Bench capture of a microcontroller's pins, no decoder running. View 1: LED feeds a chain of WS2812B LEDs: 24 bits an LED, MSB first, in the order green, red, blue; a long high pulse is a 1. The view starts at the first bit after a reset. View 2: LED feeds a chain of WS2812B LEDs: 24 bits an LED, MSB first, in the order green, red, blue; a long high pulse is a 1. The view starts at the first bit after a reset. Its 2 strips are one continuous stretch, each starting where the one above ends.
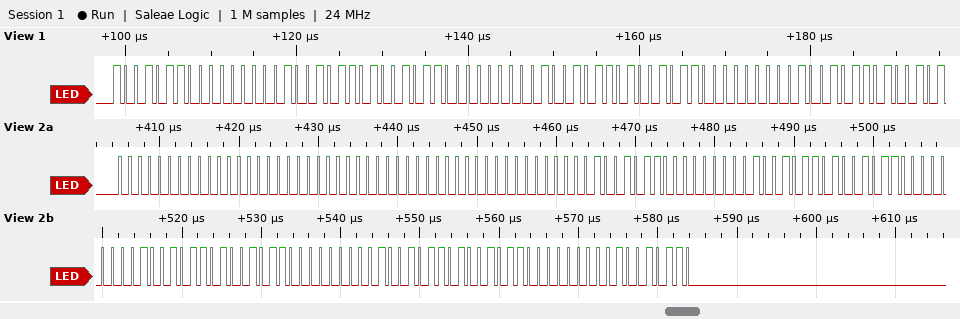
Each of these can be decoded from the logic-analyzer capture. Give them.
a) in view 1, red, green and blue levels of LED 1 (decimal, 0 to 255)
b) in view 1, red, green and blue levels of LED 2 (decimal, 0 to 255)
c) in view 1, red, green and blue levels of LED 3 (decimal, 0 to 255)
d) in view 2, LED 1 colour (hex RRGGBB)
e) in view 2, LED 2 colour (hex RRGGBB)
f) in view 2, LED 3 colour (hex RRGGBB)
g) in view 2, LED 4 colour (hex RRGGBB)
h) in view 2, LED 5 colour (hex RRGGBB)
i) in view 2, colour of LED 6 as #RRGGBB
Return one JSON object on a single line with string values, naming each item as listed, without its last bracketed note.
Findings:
{"in view 1, red, green and blue levels of LED 1": "0, 150, 150", "in view 1, red, green and blue levels of LED 2": "0, 150, 150", "in view 1, red, green and blue levels of LED 3": "0, 150, 150", "in view 2, LED 1 colour": "#000000", "in view 2, LED 2 colour": "#000000", "in view 2, LED 3 colour": "#009696", "in view 2, LED 4 colour": "#009696", "in view 2, LED 5 colour": "#009696", "in view 2, colour of LED 6 as #RRGGBB": "#009696"}
